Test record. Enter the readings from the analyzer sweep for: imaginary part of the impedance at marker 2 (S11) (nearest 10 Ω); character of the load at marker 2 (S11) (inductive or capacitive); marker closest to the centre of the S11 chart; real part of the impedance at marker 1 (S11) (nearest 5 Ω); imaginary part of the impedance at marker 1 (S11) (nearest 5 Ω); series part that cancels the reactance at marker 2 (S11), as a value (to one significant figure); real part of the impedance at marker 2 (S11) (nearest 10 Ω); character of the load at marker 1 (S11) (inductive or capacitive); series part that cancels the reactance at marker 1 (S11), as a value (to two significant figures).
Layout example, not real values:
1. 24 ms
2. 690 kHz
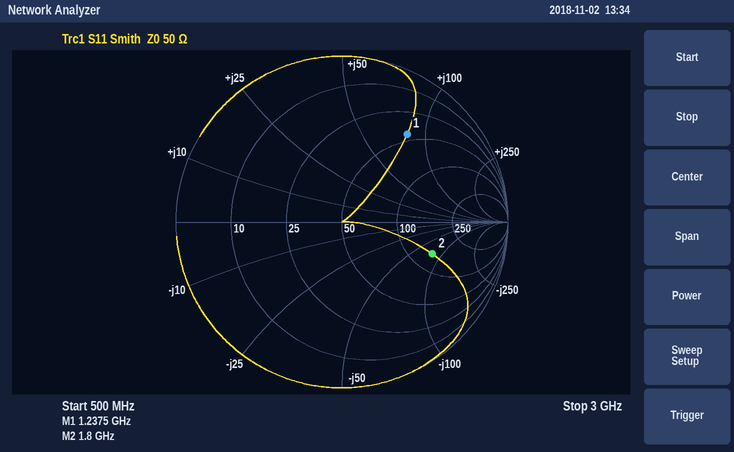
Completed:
1. -80 Ω
2. capacitive
3. marker 2
4. 45 Ω
5. +80 Ω
6. 7 nH
7. 140 Ω
8. inductive
9. 1.6 pF
